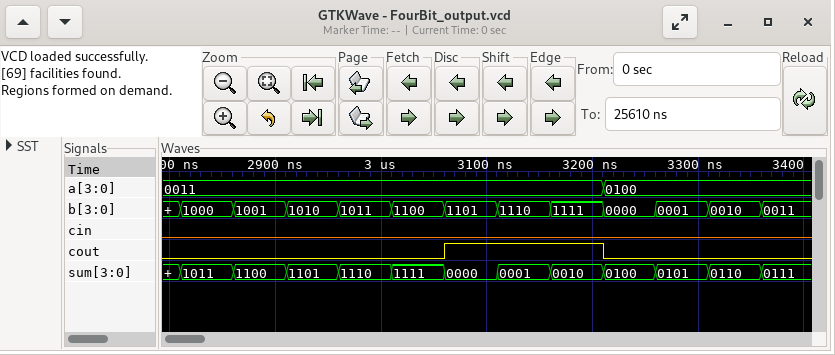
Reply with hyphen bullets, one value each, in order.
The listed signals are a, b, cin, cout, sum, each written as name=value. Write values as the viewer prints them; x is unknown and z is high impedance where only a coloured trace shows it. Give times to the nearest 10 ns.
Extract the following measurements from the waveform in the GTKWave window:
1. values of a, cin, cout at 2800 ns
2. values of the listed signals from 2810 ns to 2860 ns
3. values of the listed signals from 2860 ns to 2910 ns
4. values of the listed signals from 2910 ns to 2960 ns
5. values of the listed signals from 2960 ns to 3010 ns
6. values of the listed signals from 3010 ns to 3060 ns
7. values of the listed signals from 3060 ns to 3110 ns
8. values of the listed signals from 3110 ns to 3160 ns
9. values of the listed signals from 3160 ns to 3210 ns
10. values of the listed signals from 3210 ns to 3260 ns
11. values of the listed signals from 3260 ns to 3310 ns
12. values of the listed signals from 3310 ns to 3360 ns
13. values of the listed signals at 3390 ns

- a=0011, cin=0, cout=0
- a=0011, b=1000, cin=0, cout=0, sum=1011
- a=0011, b=1001, cin=0, cout=0, sum=1100
- a=0011, b=1010, cin=0, cout=0, sum=1101
- a=0011, b=1011, cin=0, cout=0, sum=1110
- a=0011, b=1100, cin=0, cout=0, sum=1111
- a=0011, b=1101, cin=0, cout=1, sum=0000
- a=0011, b=1110, cin=0, cout=1, sum=0001
- a=0011, b=1111, cin=0, cout=1, sum=0010
- a=0100, b=0000, cin=0, cout=0, sum=0100
- a=0100, b=0001, cin=0, cout=0, sum=0101
- a=0100, b=0010, cin=0, cout=0, sum=0110
- a=0100, b=0011, cin=0, cout=0, sum=0111
